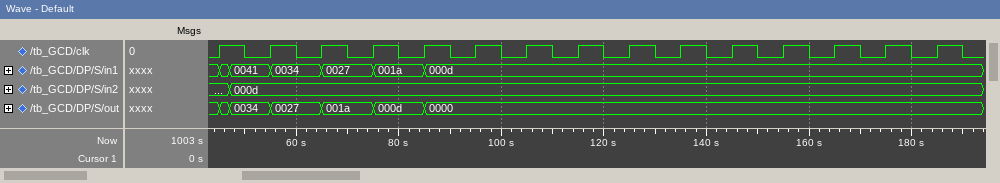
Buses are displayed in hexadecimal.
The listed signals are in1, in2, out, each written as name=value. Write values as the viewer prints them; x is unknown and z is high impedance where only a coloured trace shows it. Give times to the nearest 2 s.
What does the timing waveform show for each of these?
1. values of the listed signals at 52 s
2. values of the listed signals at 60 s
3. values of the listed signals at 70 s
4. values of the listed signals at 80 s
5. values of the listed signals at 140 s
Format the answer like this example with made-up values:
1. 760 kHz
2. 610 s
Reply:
1. in1=0041, in2=000d, out=0034
2. in1=0034, in2=000d, out=0027
3. in1=0027, in2=000d, out=001a
4. in1=001a, in2=000d, out=000d
5. in1=000d, in2=000d, out=0000
